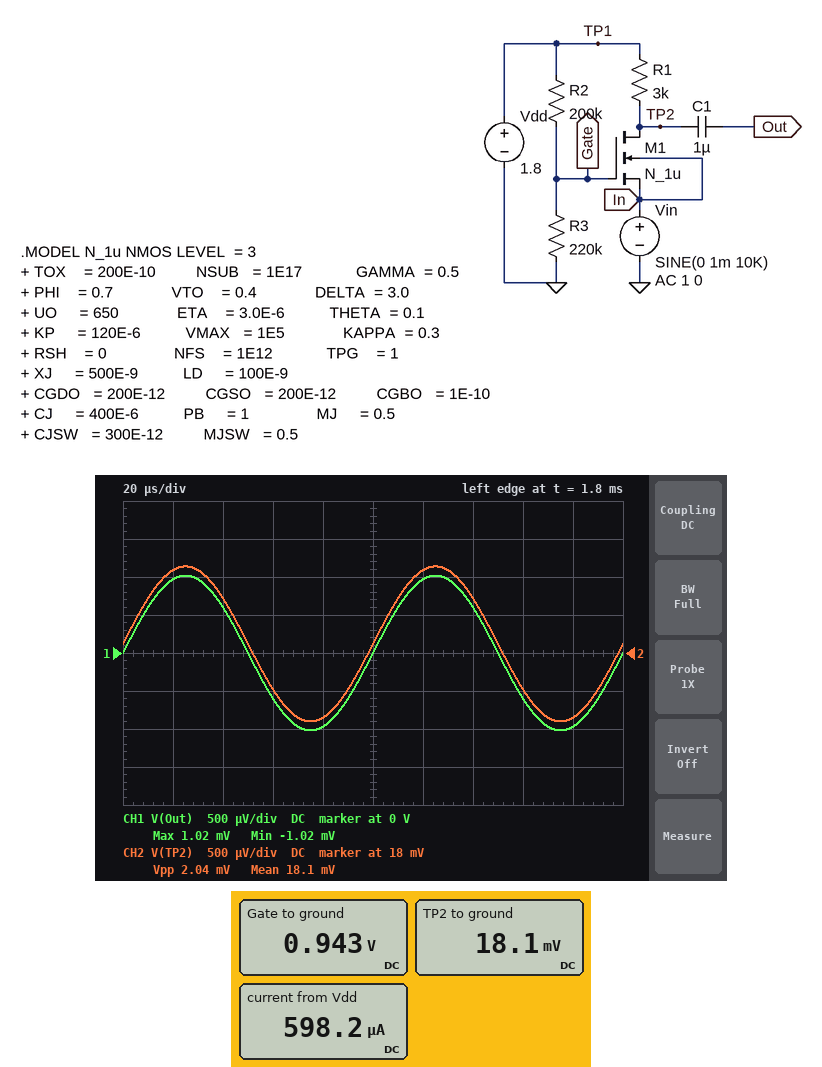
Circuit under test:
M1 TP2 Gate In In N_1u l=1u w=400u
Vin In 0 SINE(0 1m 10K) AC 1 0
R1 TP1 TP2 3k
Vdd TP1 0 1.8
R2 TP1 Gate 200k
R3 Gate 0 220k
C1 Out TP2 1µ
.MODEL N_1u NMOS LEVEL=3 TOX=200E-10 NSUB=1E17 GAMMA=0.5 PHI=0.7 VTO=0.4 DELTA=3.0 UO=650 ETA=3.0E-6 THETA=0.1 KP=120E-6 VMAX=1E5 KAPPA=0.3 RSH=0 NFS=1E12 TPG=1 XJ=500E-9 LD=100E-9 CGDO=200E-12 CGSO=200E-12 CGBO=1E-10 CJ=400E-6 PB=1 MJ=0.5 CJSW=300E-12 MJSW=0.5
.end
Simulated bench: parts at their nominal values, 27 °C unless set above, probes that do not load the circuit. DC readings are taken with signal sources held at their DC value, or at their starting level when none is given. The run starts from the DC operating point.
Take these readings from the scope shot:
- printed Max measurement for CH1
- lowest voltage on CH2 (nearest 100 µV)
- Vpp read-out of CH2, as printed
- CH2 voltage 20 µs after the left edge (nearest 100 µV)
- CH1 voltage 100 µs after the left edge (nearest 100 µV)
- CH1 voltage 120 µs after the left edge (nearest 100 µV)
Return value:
1.02 mV
17.1 mV
2.04 mV
19.1 mV
0 V
1.0 mV
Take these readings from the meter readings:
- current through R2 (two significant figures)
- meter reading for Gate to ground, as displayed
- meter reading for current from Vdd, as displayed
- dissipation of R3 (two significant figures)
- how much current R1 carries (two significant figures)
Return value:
4.3 µA
0.943 V
598.2 µA
4.0 µW
590 µA
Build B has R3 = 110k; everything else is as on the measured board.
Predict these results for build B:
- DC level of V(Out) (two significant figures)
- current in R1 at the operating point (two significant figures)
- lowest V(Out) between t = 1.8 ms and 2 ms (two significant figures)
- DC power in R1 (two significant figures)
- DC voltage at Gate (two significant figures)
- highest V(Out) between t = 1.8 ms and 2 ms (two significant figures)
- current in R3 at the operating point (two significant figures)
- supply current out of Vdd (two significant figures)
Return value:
38 mV
590 µA
-1.1 mV
1.0 mW
640 mV
1.1 mV
5.8 µA
590 µA
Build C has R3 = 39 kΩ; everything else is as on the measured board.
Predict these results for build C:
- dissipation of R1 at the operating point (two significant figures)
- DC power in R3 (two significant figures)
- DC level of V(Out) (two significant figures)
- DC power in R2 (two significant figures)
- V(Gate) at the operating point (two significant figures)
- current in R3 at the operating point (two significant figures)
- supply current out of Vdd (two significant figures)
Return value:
470 nW
2.2 µW
1.8 V
11 µW
290 mV
7.5 µA
20 µA
